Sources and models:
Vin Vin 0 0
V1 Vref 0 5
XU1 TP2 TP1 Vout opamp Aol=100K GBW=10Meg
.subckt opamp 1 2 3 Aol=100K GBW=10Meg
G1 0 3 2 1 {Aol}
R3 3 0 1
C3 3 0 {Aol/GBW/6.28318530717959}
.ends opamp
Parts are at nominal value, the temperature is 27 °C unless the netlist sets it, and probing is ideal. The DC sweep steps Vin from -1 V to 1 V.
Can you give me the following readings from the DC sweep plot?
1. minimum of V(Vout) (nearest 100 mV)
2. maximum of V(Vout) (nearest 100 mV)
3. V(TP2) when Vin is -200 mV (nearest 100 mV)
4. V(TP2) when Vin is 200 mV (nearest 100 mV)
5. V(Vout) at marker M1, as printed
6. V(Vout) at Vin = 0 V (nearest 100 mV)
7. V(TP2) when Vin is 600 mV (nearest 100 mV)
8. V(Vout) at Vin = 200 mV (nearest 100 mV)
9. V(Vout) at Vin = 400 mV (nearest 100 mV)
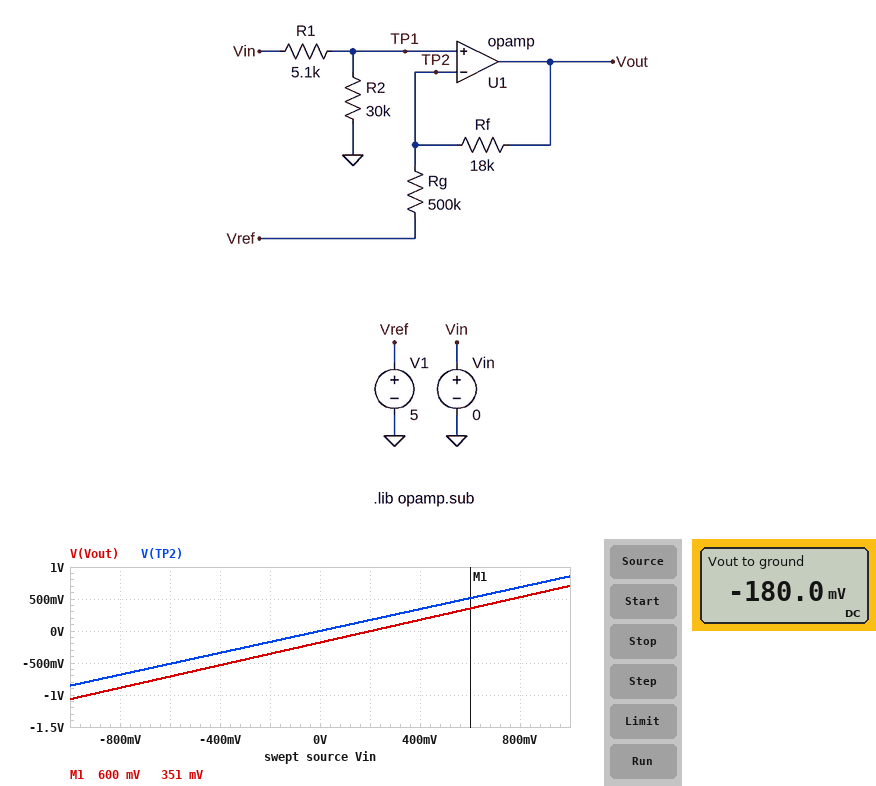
-1.1 V
700 mV
-200 mV
200 mV
351 mV
-200 mV
500 mV
0 V
200 mV
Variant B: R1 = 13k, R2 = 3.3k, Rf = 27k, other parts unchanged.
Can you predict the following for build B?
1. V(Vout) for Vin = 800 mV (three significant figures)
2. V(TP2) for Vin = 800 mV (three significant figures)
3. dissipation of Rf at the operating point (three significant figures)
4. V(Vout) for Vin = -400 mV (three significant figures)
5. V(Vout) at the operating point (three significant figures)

-99.3 mV
162 mV
2.70 µW
-355 mV
-270 mV
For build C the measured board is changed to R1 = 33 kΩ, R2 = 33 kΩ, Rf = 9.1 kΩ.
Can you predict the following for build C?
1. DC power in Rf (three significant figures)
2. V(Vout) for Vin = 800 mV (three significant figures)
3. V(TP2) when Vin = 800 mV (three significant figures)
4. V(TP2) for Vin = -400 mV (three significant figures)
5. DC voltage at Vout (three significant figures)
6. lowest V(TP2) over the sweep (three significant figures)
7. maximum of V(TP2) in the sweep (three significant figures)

910 nW
316 mV
400 mV
-200 mV
-91.0 mV
-500 mV
500 mV
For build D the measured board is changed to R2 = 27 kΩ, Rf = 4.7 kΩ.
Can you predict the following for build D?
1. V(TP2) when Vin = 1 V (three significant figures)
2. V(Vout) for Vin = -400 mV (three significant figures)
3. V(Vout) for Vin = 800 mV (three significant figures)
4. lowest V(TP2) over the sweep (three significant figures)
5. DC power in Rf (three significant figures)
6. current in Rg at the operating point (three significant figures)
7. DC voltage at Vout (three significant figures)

841 mV
-387 mV
632 mV
-841 mV
470 nW
10.0 µA
-47.0 mV
